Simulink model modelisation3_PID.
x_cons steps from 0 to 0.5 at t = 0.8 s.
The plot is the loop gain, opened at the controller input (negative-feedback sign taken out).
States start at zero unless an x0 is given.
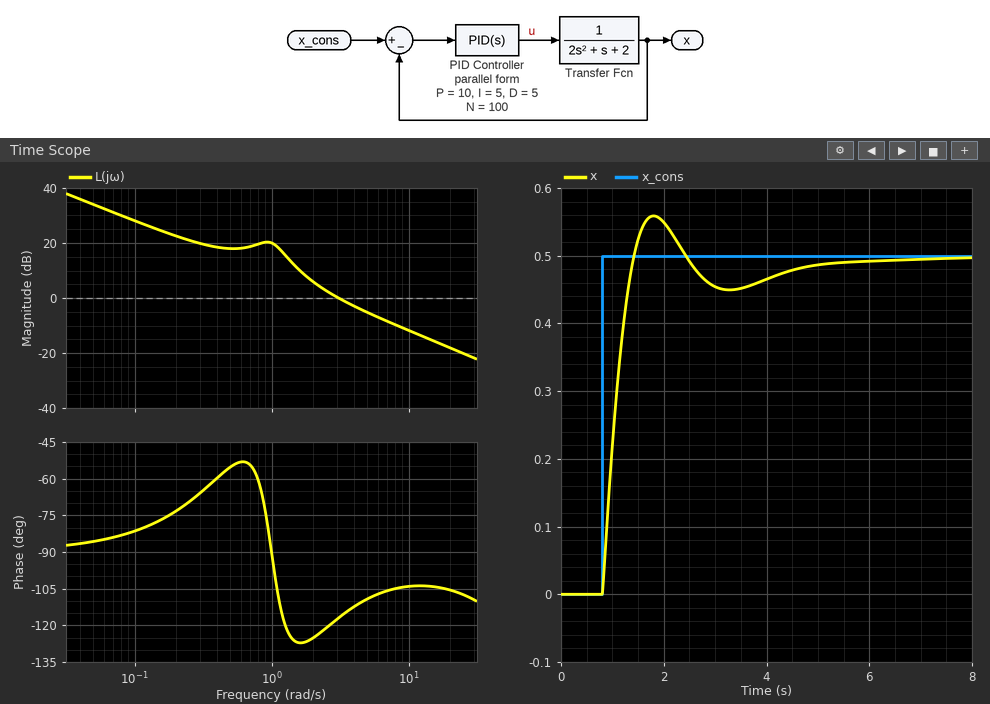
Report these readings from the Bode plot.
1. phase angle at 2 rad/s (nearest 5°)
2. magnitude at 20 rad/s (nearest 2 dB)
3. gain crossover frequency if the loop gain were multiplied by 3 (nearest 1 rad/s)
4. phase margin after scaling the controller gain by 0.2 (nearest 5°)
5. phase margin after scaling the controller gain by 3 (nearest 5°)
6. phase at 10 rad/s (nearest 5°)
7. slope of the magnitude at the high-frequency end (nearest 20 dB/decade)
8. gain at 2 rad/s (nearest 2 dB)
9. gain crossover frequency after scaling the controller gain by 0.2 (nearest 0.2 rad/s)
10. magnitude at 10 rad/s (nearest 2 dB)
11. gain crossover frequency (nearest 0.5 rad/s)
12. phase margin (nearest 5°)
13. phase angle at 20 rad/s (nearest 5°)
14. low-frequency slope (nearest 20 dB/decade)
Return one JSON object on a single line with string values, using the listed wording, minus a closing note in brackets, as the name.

{"phase angle at 2 rad/s": "-125°", "magnitude at 20 rad/s": "-18 dB", "gain crossover frequency if the loop gain were multiplied by 3": "8 rad/s", "phase margin after scaling the controller gain by 0.2": "55°", "phase margin after scaling the controller gain by 3": "75°", "phase at 10 rad/s": "-105°", "slope of the magnitude at the high-frequency end": "-20 dB/decade", "gain at 2 rad/s": "6 dB", "gain crossover frequency after scaling the controller gain by 0.2": "1.4 rad/s", "magnitude at 10 rad/s": "-12 dB", "gain crossover frequency": "3.0 rad/s", "phase margin": "65°", "phase angle at 20 rad/s": "-105°", "low-frequency slope": "-20 dB/decade"}
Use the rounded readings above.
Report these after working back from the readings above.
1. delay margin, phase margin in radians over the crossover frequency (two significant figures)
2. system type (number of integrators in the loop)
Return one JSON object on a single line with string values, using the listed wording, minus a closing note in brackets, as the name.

{"delay margin, phase margin in radians over the crossover frequency": "0.38 s", "system type": "1"}
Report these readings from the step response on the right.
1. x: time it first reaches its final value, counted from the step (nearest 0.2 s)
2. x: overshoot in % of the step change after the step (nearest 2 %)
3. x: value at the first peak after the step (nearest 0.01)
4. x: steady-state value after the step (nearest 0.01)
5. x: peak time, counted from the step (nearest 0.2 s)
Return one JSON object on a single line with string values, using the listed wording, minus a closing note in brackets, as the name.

{"x: time it first reaches its final value, counted from the step": "0.6 s", "x: overshoot in % of the step change after the step": "12 %", "x: value at the first peak after the step": "0.56", "x: steady-state value after the step": "0.50", "x: peak time, counted from the step": "1.0 s"}
